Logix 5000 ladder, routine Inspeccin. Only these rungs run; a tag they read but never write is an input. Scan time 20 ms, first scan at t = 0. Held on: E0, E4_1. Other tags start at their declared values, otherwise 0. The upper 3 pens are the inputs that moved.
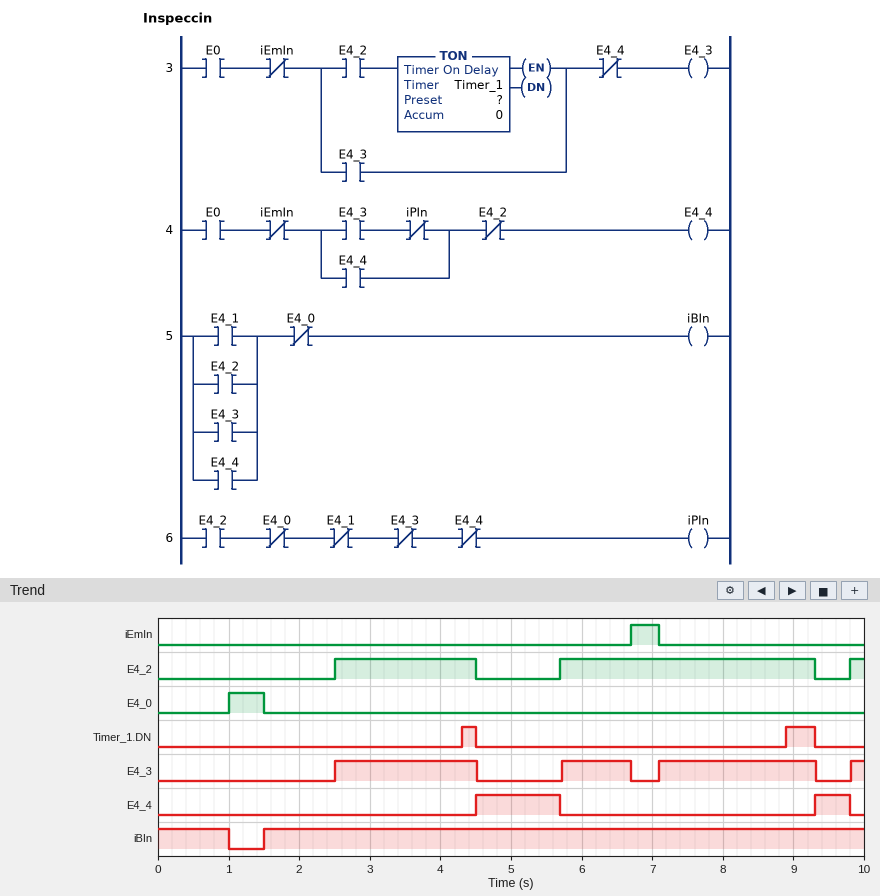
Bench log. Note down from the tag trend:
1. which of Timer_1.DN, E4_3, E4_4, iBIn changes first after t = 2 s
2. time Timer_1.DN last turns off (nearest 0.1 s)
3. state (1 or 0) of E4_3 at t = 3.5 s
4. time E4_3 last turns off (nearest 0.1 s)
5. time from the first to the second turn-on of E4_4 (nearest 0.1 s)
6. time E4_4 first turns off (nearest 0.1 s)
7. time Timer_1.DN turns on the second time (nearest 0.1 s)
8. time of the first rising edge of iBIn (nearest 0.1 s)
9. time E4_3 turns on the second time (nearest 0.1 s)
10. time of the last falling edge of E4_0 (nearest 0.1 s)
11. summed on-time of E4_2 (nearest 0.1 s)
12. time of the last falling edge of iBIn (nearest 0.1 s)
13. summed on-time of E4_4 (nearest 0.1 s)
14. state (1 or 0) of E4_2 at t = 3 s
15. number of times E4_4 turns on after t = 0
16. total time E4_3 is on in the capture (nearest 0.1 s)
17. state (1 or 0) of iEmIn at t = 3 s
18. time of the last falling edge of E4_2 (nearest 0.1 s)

E4_3
9.3 s
1
9.3 s
4.8 s
5.7 s
8.9 s
1.5 s
5.7 s
1.5 s
5.8 s
1.0 s
1.7 s
1
2
5.4 s
0
9.3 s
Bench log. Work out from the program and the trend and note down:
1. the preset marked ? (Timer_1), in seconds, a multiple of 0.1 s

1.8 s
